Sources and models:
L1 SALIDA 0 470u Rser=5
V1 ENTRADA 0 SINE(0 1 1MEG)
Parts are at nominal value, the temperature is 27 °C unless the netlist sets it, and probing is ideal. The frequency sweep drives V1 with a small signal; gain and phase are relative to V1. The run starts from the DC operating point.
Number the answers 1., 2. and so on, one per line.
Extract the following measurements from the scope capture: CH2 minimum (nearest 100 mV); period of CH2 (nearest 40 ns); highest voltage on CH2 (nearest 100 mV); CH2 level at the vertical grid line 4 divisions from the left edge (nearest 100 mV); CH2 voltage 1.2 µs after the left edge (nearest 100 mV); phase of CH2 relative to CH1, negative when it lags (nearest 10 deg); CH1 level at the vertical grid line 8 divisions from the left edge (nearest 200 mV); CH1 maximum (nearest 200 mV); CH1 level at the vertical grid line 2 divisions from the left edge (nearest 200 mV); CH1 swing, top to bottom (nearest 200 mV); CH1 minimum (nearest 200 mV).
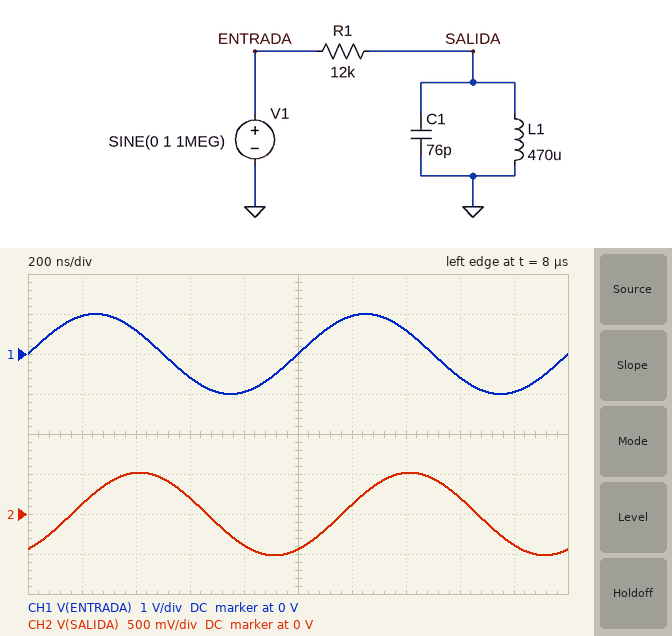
1. -500 mV
2. 1.00 µs
3. 500 mV
4. -400 mV
5. 100 mV
6. -60 deg
7. -600 mV
8. 1.0 V
9. 600 mV
10. 2.0 V
11. -1.0 V
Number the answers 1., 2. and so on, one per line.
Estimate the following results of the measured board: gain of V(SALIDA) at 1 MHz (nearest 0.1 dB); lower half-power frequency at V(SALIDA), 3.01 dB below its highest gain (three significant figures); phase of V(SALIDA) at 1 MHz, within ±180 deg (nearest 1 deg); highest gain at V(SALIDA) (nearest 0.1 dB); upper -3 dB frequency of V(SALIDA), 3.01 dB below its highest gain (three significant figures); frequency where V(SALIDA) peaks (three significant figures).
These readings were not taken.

1. -5.8 dB
2. 759 kHz
3. -59 deg
4. -0.1 dB
5. 935 kHz
6. 842 kHz
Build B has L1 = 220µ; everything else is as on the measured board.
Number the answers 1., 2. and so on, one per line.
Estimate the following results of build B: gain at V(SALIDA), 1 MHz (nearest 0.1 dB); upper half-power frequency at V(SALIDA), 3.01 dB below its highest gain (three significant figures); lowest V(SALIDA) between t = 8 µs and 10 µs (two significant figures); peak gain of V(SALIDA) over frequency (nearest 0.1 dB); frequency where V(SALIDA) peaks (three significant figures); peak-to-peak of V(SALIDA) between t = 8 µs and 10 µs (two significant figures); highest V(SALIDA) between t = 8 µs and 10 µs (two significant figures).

1. -9.9 dB
2. 1.32 MHz
3. -320 mV
4. -0.2 dB
5. 1.23 MHz
6. 640 mV
7. 320 mV
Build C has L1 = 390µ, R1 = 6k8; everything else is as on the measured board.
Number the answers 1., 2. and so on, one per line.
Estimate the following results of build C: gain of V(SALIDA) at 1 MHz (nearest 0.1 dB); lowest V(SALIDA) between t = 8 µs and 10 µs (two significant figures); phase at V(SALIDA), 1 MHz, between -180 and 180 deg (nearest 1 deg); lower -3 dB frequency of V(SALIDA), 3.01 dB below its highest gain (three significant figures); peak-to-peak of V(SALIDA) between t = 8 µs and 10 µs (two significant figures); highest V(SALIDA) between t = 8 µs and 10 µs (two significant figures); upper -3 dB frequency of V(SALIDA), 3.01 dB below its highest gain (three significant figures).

1. -0.9 dB
2. -900 mV
3. -25 deg
4. 783 kHz
5. 1.8 V
6. 900 mV
7. 1.09 MHz
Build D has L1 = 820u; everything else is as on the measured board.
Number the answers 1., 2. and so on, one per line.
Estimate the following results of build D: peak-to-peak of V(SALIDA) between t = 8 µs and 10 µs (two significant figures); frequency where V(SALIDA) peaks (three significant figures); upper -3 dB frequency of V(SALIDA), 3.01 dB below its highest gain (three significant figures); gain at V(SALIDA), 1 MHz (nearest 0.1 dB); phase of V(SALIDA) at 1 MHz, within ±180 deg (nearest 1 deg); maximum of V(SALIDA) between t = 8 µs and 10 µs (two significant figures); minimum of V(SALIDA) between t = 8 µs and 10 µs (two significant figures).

1. 570 mV
2. 638 kHz
3. 731 kHz
4. -11.0 dB
5. -74 deg
6. 280 mV
7. -280 mV
